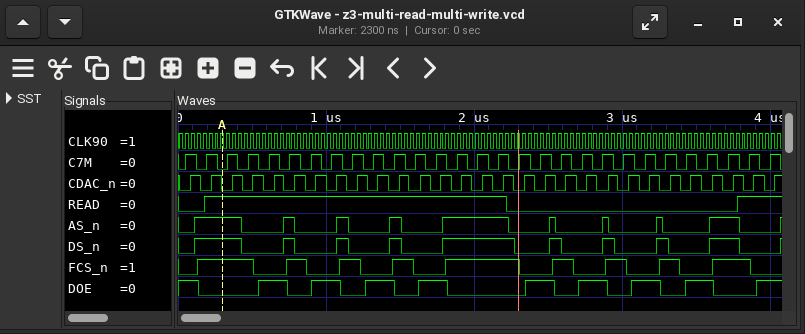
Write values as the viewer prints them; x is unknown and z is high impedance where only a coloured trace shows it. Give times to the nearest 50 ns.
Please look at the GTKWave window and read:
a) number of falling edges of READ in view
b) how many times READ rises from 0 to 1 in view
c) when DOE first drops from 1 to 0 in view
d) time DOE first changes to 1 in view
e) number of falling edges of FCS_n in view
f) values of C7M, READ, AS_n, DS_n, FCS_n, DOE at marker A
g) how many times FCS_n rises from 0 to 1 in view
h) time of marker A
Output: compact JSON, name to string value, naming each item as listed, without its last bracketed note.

{"number of falling edges of READ in view": "1", "how many times READ rises from 0 to 1 in view": "2", "when DOE first drops from 1 to 0 in view": "150 ns", "time DOE first changes to 1 in view": "550 ns", "number of falling edges of FCS_n in view": "9", "values of C7M, READ, AS_n, DS_n, FCS_n, DOE at marker A": "C7M=0, READ=1, AS_n=1, DS_n=1, FCS_n=1, DOE=0", "how many times FCS_n rises from 0 to 1 in view": "9", "time of marker A": "300 ns"}
